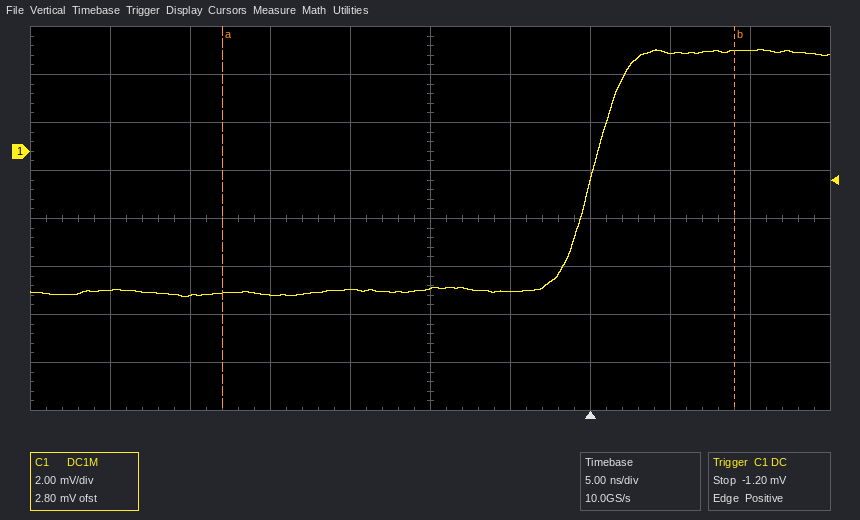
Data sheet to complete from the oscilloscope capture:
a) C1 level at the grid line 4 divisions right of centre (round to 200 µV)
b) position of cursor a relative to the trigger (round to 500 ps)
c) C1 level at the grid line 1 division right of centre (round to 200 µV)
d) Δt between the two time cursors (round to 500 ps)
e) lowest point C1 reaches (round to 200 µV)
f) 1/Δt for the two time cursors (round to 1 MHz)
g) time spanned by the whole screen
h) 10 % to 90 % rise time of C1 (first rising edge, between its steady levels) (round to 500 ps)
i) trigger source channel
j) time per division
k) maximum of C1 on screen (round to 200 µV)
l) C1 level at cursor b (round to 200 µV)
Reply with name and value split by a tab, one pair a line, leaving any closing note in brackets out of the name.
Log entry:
C1 level at the grid line 4 divisions right of centre	4.2 mV
position of cursor a relative to the trigger	-23.0 ns
C1 level at the grid line 1 division right of centre	-5.8 mV
Δt between the two time cursors	32.0 ns
lowest point C1 reaches	-6.0 mV
1/Δt for the two time cursors	31 MHz
time spanned by the whole screen	50 ns
10 % to 90 % rise time of C1 (first rising edge, between its steady levels)	4.0 ns
trigger source channel	C1
time per division	5 ns
maximum of C1 on screen	4.2 mV
C1 level at cursor b	4.2 mV
